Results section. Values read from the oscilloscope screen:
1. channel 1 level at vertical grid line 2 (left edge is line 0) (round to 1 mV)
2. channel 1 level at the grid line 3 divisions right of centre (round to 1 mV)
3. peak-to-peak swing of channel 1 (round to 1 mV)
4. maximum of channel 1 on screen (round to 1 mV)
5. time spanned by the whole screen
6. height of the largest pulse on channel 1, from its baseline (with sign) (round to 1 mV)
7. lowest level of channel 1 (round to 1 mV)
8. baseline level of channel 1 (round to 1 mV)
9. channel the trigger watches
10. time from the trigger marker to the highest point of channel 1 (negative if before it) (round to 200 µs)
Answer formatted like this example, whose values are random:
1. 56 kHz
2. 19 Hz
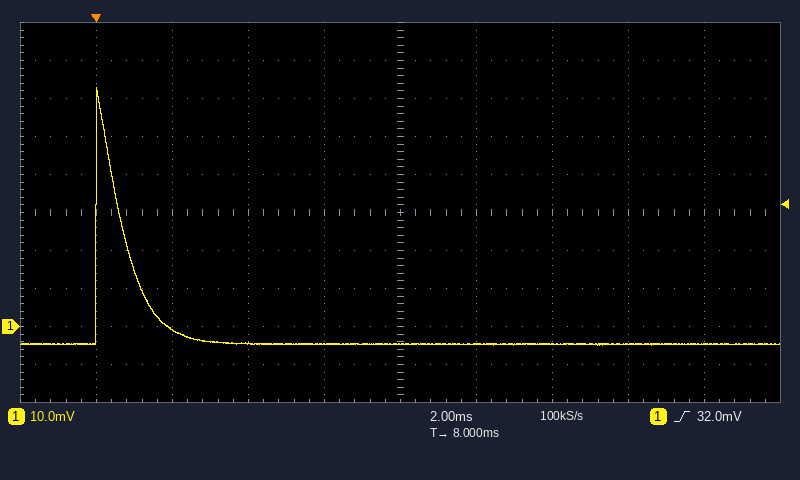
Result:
1. -1 mV
2. -5 mV
3. 68 mV
4. 63 mV
5. 20 ms
6. +68 mV
7. -5 mV
8. -5 mV
9. channel 1
10. 0.0 ms
